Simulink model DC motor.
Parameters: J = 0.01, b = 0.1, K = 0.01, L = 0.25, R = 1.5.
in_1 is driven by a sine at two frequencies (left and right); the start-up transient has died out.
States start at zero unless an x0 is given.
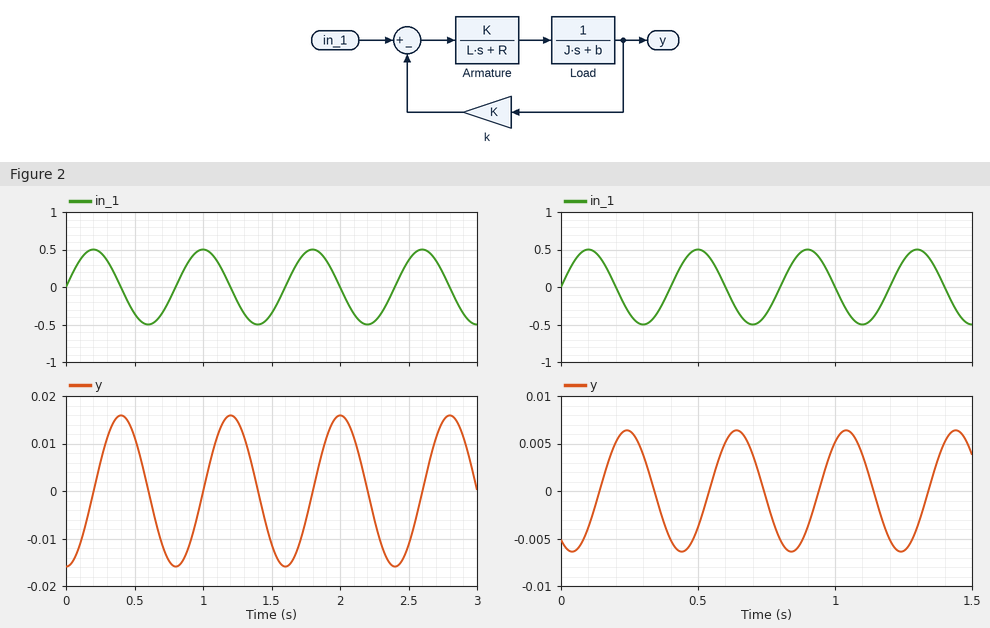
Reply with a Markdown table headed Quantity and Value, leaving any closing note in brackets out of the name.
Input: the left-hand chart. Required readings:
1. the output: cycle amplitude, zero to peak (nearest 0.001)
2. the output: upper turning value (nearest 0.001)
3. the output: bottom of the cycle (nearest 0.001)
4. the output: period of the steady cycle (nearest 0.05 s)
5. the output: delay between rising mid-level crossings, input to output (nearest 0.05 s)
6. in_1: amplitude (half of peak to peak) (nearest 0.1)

| Quantity | Value |
|---|---|
| the output: cycle amplitude, zero to peak | 0.016 |
| the output: upper turning value | 0.016 |
| the output: bottom of the cycle | -0.016 |
| the output: period of the steady cycle | 0.80 s |
| the output: delay between rising mid-level crossings, input to output | 0.20 s |
| in_1: amplitude (half of peak to peak) | 0.5 |
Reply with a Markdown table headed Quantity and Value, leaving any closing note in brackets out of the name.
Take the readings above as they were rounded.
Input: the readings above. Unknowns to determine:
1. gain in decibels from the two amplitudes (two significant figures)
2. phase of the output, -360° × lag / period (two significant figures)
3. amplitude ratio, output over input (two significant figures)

| Quantity | Value |
|---|---|
| gain in decibels from the two amplitudes | -30 dB |
| phase of the output, -360° × lag / period | -90° |
| amplitude ratio, output over input | 0.032 |
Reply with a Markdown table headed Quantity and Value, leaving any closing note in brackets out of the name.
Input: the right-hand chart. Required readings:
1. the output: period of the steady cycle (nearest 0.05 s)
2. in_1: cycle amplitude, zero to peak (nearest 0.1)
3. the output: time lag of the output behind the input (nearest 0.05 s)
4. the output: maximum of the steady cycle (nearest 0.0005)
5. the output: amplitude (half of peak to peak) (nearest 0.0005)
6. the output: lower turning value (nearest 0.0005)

| Quantity | Value |
|---|---|
| the output: period of the steady cycle | 0.40 s |
| in_1: cycle amplitude, zero to peak | 0.5 |
| the output: time lag of the output behind the input | 0.15 s |
| the output: maximum of the steady cycle | 0.0065 |
| the output: amplitude (half of peak to peak) | 0.0065 |
| the output: lower turning value | -0.0065 |
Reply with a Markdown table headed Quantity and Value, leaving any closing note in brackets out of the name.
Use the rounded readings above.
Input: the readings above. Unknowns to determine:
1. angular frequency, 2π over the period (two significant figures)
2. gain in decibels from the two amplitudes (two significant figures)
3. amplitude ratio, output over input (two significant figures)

| Quantity | Value |
|---|---|
| angular frequency, 2π over the period | 16 rad/s |
| gain in decibels from the two amplitudes | -38 dB |
| amplitude ratio, output over input | 0.013 |
